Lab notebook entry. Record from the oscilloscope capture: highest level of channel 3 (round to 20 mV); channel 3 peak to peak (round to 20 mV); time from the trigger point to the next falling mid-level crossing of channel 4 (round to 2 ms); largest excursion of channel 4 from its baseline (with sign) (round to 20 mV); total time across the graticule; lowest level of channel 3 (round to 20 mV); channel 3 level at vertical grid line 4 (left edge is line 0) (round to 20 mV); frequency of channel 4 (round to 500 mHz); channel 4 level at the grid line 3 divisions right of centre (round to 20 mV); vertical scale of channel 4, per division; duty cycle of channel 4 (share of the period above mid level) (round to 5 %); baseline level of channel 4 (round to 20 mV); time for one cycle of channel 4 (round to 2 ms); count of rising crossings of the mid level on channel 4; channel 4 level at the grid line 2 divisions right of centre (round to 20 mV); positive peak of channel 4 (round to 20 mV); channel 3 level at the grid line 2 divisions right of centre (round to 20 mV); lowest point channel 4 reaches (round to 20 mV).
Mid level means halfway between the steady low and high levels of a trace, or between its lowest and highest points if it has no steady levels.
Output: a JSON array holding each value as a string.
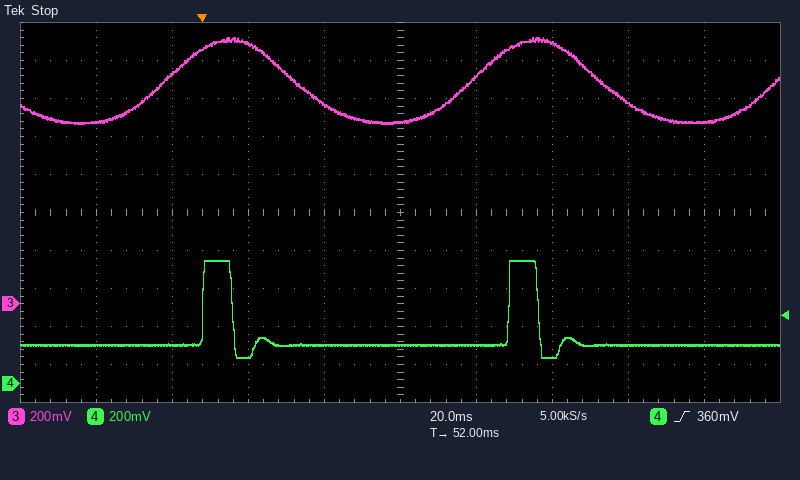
["1.40 V", "460 mV", "8 ms", "+440 mV", "200 ms", "940 mV", "1.06 V", "12.5 Hz", "200 mV", "200 mV", "10 %", "200 mV", "80 ms", "2", "140 mV", "640 mV", "1.38 V", "140 mV"]
